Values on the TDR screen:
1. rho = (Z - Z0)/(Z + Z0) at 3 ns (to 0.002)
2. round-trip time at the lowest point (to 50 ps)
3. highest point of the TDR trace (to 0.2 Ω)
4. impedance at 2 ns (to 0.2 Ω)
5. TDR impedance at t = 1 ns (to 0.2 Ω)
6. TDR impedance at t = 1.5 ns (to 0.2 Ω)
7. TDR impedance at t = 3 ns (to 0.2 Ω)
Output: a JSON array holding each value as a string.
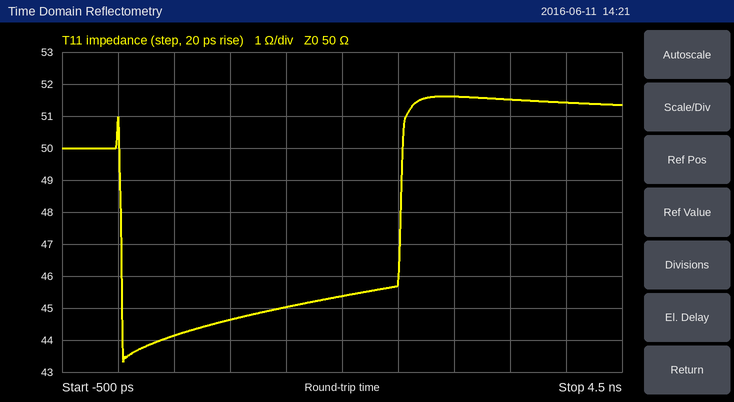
["+0.016", "50 ps", "51.6 Ω", "45.4 Ω", "44.6 Ω", "45.0 Ω", "51.6 Ω"]
